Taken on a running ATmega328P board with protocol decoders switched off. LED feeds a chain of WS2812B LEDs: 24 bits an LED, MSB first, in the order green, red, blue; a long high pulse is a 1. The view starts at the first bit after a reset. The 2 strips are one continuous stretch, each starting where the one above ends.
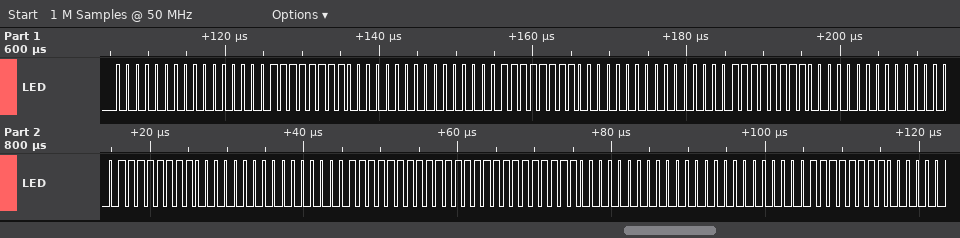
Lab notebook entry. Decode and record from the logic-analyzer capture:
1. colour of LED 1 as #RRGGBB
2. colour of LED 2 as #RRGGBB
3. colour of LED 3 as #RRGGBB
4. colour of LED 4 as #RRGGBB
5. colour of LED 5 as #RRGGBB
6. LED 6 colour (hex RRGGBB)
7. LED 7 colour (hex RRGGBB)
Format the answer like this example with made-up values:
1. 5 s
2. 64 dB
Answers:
1. #0000FF
2. #0000FF
3. #0000FF
4. #0000FF
5. #0000FF
6. #FFFF00
7. #0000FF
